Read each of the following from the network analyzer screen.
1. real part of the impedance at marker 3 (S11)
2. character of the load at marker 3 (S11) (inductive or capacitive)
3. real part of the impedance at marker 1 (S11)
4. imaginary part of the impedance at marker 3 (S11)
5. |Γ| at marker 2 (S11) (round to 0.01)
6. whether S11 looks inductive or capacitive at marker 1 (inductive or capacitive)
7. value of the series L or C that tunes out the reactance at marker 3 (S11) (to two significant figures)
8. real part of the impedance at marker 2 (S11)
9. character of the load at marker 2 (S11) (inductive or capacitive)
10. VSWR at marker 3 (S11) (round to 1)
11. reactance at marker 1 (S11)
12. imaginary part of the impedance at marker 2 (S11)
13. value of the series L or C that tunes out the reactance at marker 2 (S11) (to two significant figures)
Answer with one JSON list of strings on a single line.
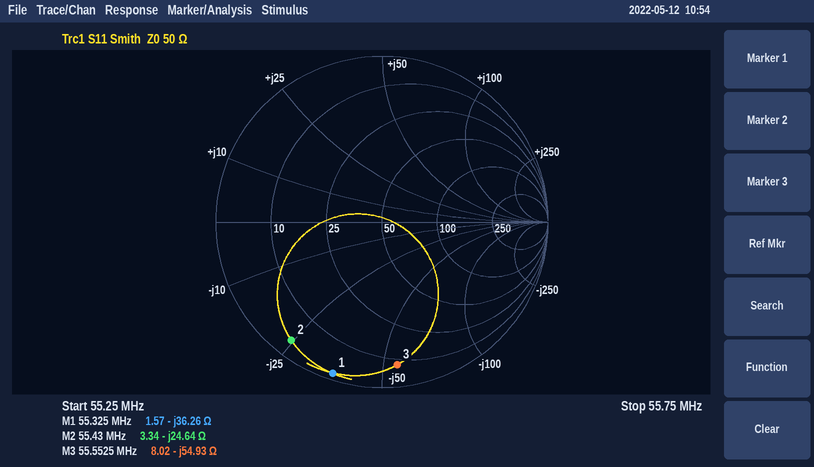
["8.02 Ω", "capacitive", "1.57 Ω", "-54.93 Ω", "0.90", "capacitive", "160 nH", "3.34 Ω", "capacitive", "14", "-36.26 Ω", "-24.64 Ω", "71 nH"]
